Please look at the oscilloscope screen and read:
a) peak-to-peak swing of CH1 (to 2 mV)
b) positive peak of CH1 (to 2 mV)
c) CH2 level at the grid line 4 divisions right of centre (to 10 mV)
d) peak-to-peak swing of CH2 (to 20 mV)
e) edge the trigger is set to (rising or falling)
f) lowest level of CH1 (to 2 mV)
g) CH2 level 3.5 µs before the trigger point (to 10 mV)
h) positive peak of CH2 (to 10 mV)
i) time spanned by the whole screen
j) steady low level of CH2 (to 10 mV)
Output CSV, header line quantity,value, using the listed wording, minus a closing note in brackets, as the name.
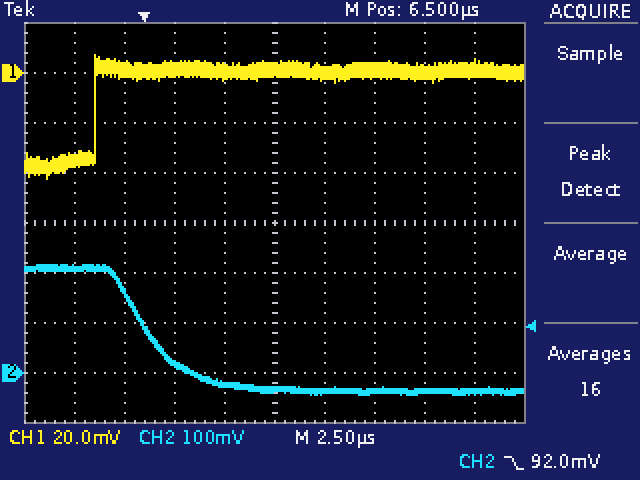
quantity,value
peak-to-peak swing of CH1,50 mV
positive peak of CH1,8 mV
CH2 level at the grid line 4 divisions right of centre,-40 mV
peak-to-peak swing of CH2,260 mV
edge the trigger is set to,falling
lowest level of CH1,-42 mV
CH2 level 3.5 µs before the trigger point,210 mV
positive peak of CH2,220 mV
time spanned by the whole screen,25 µs
steady low level of CH2,-40 mV
